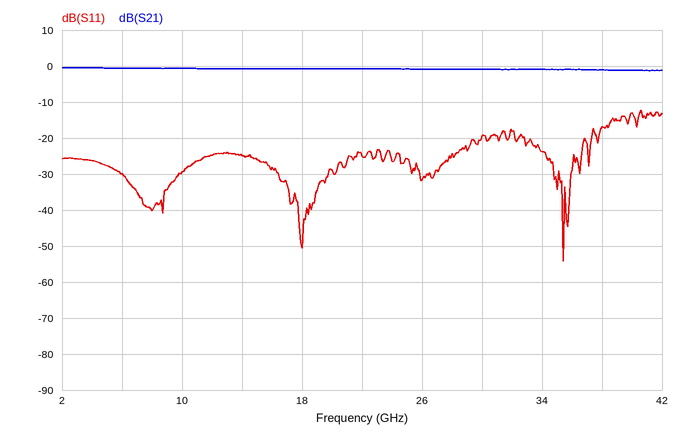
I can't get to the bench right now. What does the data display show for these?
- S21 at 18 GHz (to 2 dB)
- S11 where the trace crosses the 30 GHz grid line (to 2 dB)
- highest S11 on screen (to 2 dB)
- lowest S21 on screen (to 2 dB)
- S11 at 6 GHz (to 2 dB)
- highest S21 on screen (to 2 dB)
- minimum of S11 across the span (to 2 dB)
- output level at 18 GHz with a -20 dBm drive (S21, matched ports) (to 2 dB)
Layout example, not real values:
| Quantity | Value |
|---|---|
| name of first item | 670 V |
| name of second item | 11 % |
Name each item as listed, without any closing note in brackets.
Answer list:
| Quantity | Value |
|---|---|
| S21 at 18 GHz | 0 dB |
| S11 where the trace crosses the 30 GHz grid line | -20 dB |
| highest S11 on screen | -12 dB |
| lowest S21 on screen | -2 dB |
| S11 at 6 GHz | -30 dB |
| highest S21 on screen | 0 dB |
| minimum of S11 across the span | -54 dB |
| output level at 18 GHz with a -20 dBm drive (S21, matched ports) | -20 dBm |
